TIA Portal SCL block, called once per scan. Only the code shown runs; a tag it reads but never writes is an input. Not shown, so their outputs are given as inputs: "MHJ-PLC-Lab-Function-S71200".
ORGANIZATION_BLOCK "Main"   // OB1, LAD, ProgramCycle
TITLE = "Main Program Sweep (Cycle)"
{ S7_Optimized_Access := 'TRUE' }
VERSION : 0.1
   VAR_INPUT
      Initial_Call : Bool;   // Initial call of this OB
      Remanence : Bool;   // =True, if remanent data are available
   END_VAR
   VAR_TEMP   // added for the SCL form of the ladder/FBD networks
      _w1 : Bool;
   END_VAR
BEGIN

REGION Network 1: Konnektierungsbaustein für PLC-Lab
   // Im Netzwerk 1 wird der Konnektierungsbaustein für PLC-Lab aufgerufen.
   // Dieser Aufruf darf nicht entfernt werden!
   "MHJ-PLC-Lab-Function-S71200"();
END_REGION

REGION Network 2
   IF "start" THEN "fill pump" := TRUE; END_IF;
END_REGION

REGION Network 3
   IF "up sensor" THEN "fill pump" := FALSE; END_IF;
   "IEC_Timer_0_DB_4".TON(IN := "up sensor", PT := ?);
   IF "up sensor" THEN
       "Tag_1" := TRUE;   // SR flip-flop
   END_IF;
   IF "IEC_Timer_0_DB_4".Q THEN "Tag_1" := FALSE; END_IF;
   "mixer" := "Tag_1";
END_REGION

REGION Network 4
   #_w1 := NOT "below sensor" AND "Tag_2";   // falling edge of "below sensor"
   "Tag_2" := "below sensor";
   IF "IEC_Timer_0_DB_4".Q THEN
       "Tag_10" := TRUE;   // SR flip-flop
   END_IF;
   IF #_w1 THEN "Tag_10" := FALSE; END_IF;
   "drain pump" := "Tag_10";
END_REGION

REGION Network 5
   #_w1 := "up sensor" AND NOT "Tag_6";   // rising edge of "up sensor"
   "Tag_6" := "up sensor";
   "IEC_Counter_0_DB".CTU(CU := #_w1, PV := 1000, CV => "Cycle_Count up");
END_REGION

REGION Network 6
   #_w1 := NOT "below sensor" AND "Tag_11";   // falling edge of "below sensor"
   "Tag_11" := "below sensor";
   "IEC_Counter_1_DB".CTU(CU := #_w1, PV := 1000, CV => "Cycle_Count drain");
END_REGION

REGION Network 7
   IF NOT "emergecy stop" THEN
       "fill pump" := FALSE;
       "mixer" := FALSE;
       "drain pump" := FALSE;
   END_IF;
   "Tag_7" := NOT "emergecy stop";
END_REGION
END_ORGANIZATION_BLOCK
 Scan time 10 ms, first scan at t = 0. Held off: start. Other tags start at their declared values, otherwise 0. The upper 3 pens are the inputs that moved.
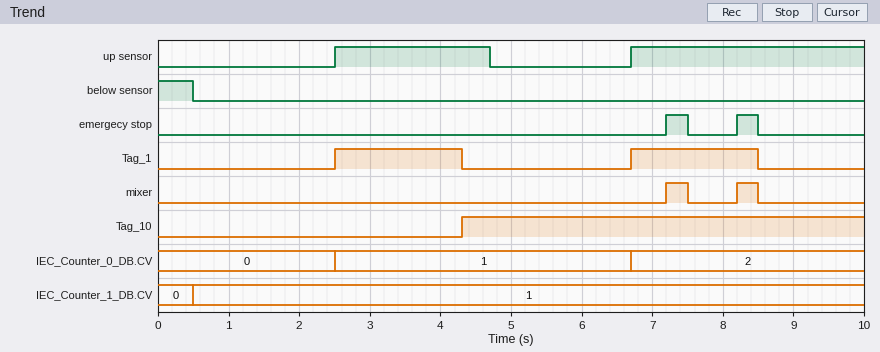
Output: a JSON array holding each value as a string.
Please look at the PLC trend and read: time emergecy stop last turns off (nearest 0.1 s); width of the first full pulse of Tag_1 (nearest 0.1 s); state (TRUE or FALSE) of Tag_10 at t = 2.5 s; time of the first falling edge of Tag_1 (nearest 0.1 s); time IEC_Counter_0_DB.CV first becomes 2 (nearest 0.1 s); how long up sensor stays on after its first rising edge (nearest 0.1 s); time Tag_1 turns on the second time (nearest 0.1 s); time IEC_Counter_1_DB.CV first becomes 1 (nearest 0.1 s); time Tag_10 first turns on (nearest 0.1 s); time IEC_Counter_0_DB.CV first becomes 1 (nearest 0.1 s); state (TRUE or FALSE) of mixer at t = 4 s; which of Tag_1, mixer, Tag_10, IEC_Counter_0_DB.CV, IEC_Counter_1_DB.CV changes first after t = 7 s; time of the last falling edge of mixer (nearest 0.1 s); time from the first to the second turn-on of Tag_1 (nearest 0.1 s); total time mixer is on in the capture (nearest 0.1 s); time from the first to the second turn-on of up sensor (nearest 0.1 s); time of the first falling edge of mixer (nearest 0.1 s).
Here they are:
["8.5 s", "1.8 s", "FALSE", "4.3 s", "6.7 s", "2.2 s", "6.7 s", "0.5 s", "4.3 s", "2.5 s", "FALSE", "mixer", "8.5 s", "4.2 s", "0.6 s", "4.2 s", "7.5 s"]
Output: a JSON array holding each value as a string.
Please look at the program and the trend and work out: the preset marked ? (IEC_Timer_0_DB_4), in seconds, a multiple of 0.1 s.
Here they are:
["1.8 s"]
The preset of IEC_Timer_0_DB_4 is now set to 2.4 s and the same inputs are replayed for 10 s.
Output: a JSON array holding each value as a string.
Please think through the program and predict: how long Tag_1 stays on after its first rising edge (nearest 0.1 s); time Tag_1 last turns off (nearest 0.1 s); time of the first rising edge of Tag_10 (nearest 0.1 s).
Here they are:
["6.6 s", "9.1 s", "9.1 s"]
